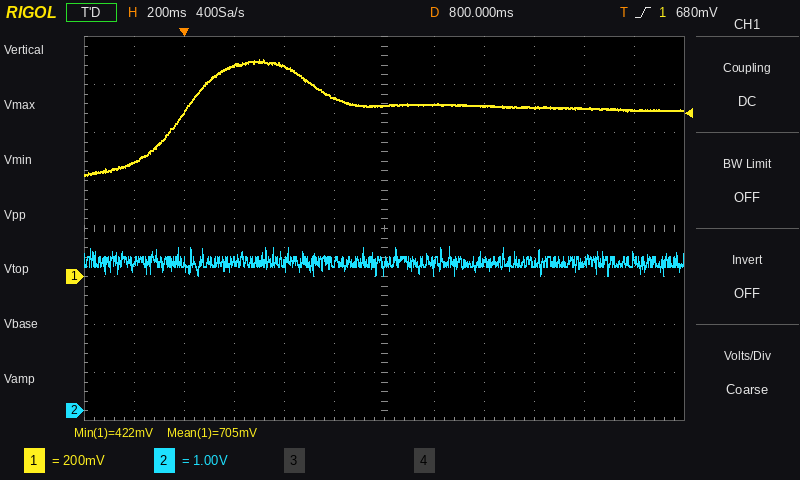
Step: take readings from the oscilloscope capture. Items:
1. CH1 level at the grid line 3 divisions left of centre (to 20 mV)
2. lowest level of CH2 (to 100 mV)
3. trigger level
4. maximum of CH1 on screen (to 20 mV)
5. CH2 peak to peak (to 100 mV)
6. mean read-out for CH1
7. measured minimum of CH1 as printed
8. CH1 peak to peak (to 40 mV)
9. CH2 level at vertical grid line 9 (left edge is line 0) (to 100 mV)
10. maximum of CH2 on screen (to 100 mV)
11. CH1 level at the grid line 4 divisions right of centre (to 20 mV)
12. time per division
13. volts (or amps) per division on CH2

880 mV
2.8 V
680 mV
900 mV
600 mV
705 mV
422 mV
480 mV
3.1 V
3.4 V
700 mV
200 ms
1 V
